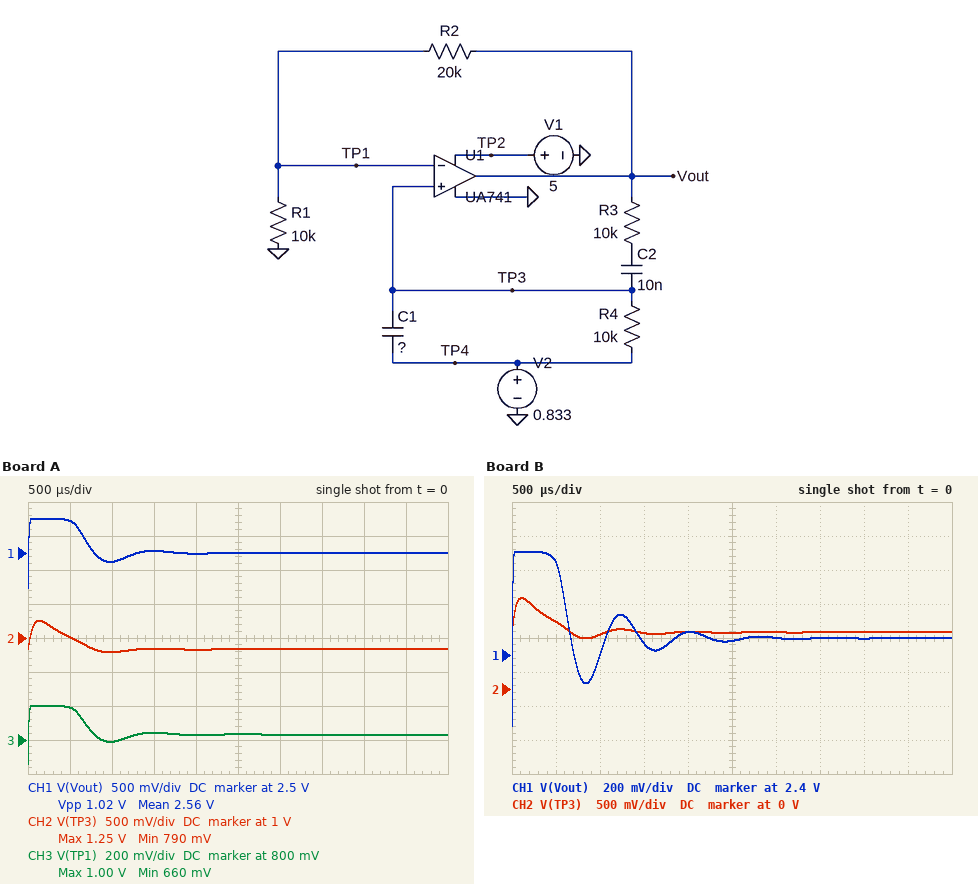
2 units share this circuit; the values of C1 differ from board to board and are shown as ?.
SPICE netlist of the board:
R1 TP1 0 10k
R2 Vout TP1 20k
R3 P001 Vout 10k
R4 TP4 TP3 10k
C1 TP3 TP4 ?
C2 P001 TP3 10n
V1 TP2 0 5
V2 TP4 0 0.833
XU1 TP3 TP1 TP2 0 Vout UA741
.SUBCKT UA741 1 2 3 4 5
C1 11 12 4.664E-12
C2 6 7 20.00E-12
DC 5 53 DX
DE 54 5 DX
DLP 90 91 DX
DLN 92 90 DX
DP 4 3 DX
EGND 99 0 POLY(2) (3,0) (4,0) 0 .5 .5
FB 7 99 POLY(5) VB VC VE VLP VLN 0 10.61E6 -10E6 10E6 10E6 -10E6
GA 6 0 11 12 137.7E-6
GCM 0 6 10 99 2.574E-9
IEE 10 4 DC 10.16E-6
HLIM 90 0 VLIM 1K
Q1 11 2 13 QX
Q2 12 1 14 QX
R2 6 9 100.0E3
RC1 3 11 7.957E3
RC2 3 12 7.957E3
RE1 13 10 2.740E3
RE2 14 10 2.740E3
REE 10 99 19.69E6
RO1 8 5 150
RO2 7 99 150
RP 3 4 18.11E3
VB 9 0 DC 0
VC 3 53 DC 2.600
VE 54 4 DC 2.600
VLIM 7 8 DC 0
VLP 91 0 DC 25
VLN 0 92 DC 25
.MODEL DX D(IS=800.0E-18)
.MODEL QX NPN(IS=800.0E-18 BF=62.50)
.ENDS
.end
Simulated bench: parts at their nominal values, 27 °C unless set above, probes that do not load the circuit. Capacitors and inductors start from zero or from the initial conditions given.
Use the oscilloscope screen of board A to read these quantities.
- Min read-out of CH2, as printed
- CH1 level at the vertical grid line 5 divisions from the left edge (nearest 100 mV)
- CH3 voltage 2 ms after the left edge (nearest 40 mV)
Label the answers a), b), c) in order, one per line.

a) 790 mV
b) 2.5 V
c) 840 mV
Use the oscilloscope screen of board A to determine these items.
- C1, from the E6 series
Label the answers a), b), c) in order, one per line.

a) 22 nF
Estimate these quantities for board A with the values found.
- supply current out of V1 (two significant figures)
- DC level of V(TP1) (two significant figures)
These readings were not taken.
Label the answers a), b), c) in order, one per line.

a) 290 µA
b) 830 mV
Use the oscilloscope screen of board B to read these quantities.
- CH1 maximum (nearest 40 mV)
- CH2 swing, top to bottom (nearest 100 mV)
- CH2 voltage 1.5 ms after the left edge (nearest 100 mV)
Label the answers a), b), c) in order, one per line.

a) 3.00 V
b) 600 mV
c) 800 mV
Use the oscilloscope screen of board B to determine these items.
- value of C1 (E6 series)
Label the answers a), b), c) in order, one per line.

a) 15 nF
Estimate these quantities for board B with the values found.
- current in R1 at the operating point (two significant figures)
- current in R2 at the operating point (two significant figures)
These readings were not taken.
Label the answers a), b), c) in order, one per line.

a) 83 µA
b) 83 µA
